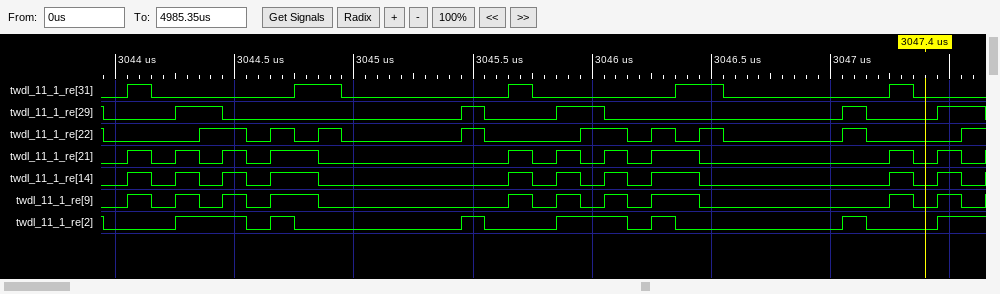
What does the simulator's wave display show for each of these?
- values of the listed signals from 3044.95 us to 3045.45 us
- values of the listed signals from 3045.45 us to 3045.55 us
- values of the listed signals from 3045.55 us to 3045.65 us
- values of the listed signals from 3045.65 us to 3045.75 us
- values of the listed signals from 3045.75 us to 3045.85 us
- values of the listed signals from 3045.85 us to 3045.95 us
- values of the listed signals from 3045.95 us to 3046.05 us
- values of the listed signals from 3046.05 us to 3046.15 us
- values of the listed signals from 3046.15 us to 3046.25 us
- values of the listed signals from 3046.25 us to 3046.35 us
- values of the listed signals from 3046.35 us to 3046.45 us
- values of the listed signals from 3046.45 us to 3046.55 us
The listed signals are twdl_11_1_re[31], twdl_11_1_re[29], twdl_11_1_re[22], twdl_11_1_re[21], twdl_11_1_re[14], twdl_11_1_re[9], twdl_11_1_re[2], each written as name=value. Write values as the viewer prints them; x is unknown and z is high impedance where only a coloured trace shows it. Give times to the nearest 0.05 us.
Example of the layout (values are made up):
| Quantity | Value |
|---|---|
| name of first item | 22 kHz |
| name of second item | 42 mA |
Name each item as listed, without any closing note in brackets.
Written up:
| Quantity | Value |
|---|---|
| values of the listed signals from 3044.95 us to 3045.45 us | twdl_11_1_re[31]=0, twdl_11_1_re[29]=0, twdl_11_1_re[22]=0, twdl_11_1_re[21]=0, twdl_11_1_re[14]=0, twdl_11_1_re[9]=0, twdl_11_1_re[2]=0 |
| values of the listed signals from 3045.45 us to 3045.55 us | twdl_11_1_re[31]=0, twdl_11_1_re[29]=1, twdl_11_1_re[22]=1, twdl_11_1_re[21]=0, twdl_11_1_re[14]=0, twdl_11_1_re[9]=0, twdl_11_1_re[2]=1 |
| values of the listed signals from 3045.55 us to 3045.65 us | twdl_11_1_re[31]=0, twdl_11_1_re[29]=0, twdl_11_1_re[22]=0, twdl_11_1_re[21]=0, twdl_11_1_re[14]=0, twdl_11_1_re[9]=0, twdl_11_1_re[2]=0 |
| values of the listed signals from 3045.65 us to 3045.75 us | twdl_11_1_re[31]=1, twdl_11_1_re[29]=0, twdl_11_1_re[22]=0, twdl_11_1_re[21]=1, twdl_11_1_re[14]=1, twdl_11_1_re[9]=1, twdl_11_1_re[2]=0 |
| values of the listed signals from 3045.75 us to 3045.85 us | twdl_11_1_re[31]=0, twdl_11_1_re[29]=0, twdl_11_1_re[22]=0, twdl_11_1_re[21]=0, twdl_11_1_re[14]=0, twdl_11_1_re[9]=0, twdl_11_1_re[2]=0 |
| values of the listed signals from 3045.85 us to 3045.95 us | twdl_11_1_re[31]=0, twdl_11_1_re[29]=1, twdl_11_1_re[22]=0, twdl_11_1_re[21]=1, twdl_11_1_re[14]=1, twdl_11_1_re[9]=1, twdl_11_1_re[2]=1 |
| values of the listed signals from 3045.95 us to 3046.05 us | twdl_11_1_re[31]=0, twdl_11_1_re[29]=1, twdl_11_1_re[22]=1, twdl_11_1_re[21]=0, twdl_11_1_re[14]=0, twdl_11_1_re[9]=0, twdl_11_1_re[2]=1 |
| values of the listed signals from 3046.05 us to 3046.15 us | twdl_11_1_re[31]=0, twdl_11_1_re[29]=0, twdl_11_1_re[22]=1, twdl_11_1_re[21]=1, twdl_11_1_re[14]=1, twdl_11_1_re[9]=1, twdl_11_1_re[2]=1 |
| values of the listed signals from 3046.15 us to 3046.25 us | twdl_11_1_re[31]=0, twdl_11_1_re[29]=0, twdl_11_1_re[22]=0, twdl_11_1_re[21]=0, twdl_11_1_re[14]=0, twdl_11_1_re[9]=0, twdl_11_1_re[2]=0 |
| values of the listed signals from 3046.25 us to 3046.35 us | twdl_11_1_re[31]=0, twdl_11_1_re[29]=0, twdl_11_1_re[22]=1, twdl_11_1_re[21]=1, twdl_11_1_re[14]=1, twdl_11_1_re[9]=1, twdl_11_1_re[2]=1 |
| values of the listed signals from 3046.35 us to 3046.45 us | twdl_11_1_re[31]=1, twdl_11_1_re[29]=0, twdl_11_1_re[22]=0, twdl_11_1_re[21]=1, twdl_11_1_re[14]=1, twdl_11_1_re[9]=1, twdl_11_1_re[2]=0 |
| values of the listed signals from 3046.45 us to 3046.55 us | twdl_11_1_re[31]=1, twdl_11_1_re[29]=0, twdl_11_1_re[22]=1, twdl_11_1_re[21]=0, twdl_11_1_re[14]=0, twdl_11_1_re[9]=0, twdl_11_1_re[2]=0 |
